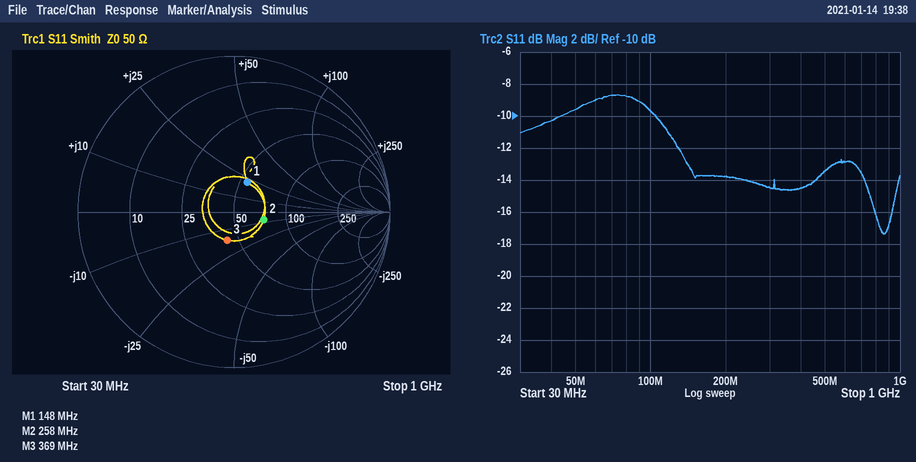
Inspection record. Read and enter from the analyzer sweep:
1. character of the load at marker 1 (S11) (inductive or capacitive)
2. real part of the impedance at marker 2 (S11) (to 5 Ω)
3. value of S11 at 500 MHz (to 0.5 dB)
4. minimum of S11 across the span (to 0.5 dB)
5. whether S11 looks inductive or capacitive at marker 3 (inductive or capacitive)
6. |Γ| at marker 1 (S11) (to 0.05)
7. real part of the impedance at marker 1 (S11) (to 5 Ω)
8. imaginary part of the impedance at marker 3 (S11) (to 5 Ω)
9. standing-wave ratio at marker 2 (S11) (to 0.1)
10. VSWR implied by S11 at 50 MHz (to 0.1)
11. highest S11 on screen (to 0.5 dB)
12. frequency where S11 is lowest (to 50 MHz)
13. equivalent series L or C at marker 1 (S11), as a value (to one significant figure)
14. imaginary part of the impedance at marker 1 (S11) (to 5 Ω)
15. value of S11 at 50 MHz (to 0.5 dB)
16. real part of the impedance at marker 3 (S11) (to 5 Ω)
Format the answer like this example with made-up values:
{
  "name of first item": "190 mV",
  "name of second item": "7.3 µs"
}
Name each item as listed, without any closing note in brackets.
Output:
{
  "character of the load at marker 1 (S11)": "inductive",
  "real part of the impedance at marker 2 (S11)": "75 Ω",
  "value of S11 at 500 MHz": "-13.5 dB",
  "minimum of S11 across the span": "-17.5 dB",
  "whether S11 looks inductive or capacitive at marker 3": "capacitive",
  "|Γ| at marker 1 (S11)": "0.20",
  "real part of the impedance at marker 1 (S11)": "55 Ω",
  "imaginary part of the impedance at marker 3 (S11)": "-15 Ω",
  "standing-wave ratio at marker 2 (S11)": "1.5",
  "VSWR implied by S11 at 50 MHz": "2.0",
  "highest S11 on screen": "-8.5 dB",
  "frequency where S11 is lowest": "850 MHz",
  "equivalent series L or C at marker 1 (S11), as a value": "20 nH",
  "imaginary part of the impedance at marker 1 (S11)": "+20 Ω",
  "value of S11 at 50 MHz": "-9.5 dB",
  "real part of the impedance at marker 3 (S11)": "45 Ω"
}
